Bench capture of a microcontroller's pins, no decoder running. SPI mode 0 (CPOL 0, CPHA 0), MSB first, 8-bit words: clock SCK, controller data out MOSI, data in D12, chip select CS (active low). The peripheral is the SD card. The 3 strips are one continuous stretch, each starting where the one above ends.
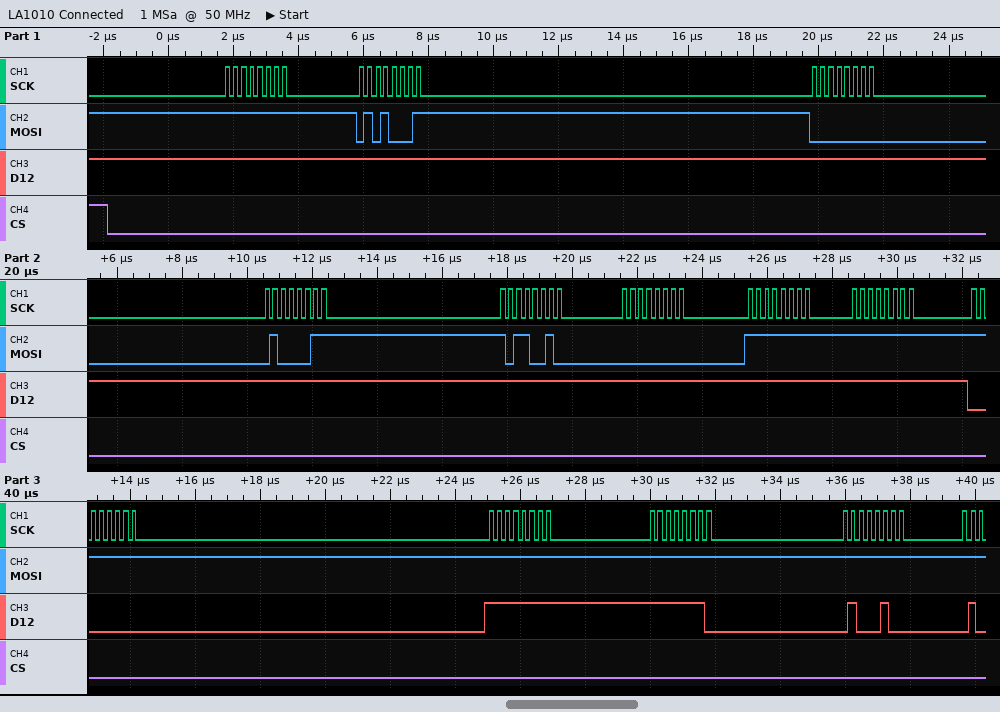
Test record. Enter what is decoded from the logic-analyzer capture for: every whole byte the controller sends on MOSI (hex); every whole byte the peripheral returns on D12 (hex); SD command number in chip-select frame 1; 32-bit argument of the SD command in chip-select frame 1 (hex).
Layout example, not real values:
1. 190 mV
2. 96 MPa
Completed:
1. FF 51 00 43 B2 00 FF FF FF FF FF FF
2. FF FF FF FF FF FF FF FF 00 FF FE 44
3. CMD17
4. 0x0043B200
